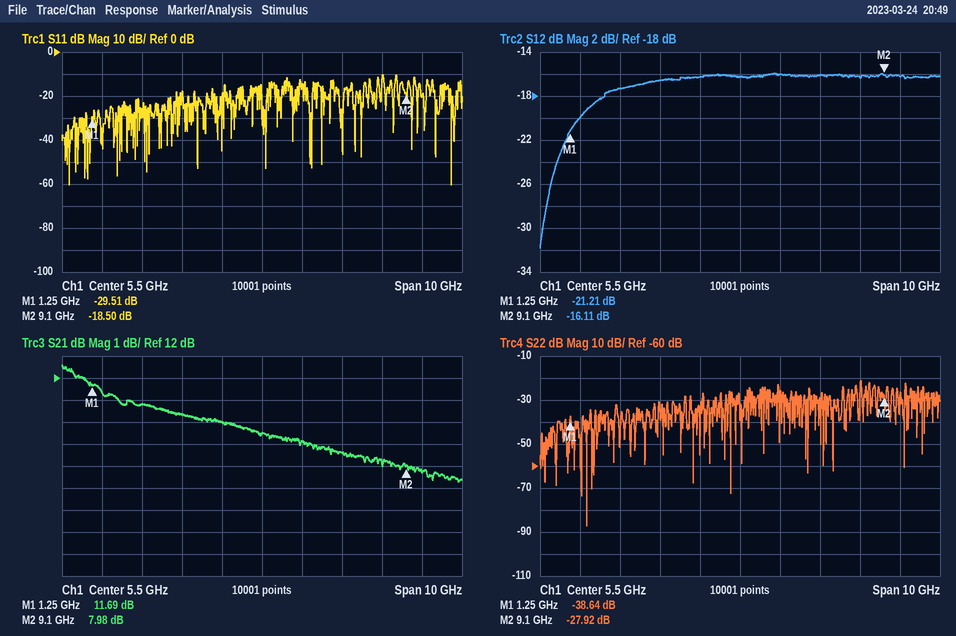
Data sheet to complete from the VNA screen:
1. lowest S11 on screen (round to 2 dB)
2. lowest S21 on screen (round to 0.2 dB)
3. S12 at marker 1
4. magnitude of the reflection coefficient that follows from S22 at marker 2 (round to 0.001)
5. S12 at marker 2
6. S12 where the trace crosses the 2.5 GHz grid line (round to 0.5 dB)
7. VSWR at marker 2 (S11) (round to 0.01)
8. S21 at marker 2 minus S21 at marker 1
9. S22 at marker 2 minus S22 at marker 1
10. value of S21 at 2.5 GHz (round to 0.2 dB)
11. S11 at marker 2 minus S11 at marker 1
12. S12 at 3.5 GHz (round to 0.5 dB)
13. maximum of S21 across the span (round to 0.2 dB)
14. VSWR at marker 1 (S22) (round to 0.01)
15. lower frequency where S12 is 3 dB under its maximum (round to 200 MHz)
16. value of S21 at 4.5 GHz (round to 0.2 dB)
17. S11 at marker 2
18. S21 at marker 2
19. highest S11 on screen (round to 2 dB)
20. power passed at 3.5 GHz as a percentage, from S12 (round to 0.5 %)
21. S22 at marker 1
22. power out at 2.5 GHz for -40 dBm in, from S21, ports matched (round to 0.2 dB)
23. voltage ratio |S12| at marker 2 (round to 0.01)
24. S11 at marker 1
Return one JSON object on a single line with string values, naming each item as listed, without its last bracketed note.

{"lowest S11 on screen": "-60 dB", "lowest S21 on screen": "7.2 dB", "S12 at marker 1": "-21.21 dB", "magnitude of the reflection coefficient that follows from S22 at marker 2": "0.040", "S12 at marker 2": "-16.11 dB", "S12 where the trace crosses the 2.5 GHz grid line": "-17.5 dB", "VSWR at marker 2 (S11)": "1.27", "S21 at marker 2 minus S21 at marker 1": "-3.71 dB", "S22 at marker 2 minus S22 at marker 1": "10.72 dB", "value of S21 at 2.5 GHz": "10.8 dB", "S11 at marker 2 minus S11 at marker 1": "11.01 dB", "S12 at 3.5 GHz": "-16.5 dB", "maximum of S21 across the span": "12.6 dB", "VSWR at marker 1 (S22)": "1.02", "lower frequency where S12 is 3 dB under its maximum": "1.8 GHz", "value of S21 at 4.5 GHz": "10.0 dB", "S11 at marker 2": "-18.50 dB", "S21 at marker 2": "7.98 dB", "highest S11 on screen": "-10 dB", "power passed at 3.5 GHz as a percentage, from S12": "2.0 %", "S22 at marker 1": "-38.64 dB", "power out at 2.5 GHz for -40 dBm in, from S21, ports matched": "-29.2 dBm", "voltage ratio |S12| at marker 2": "0.16", "S11 at marker 1": "-29.51 dB"}
